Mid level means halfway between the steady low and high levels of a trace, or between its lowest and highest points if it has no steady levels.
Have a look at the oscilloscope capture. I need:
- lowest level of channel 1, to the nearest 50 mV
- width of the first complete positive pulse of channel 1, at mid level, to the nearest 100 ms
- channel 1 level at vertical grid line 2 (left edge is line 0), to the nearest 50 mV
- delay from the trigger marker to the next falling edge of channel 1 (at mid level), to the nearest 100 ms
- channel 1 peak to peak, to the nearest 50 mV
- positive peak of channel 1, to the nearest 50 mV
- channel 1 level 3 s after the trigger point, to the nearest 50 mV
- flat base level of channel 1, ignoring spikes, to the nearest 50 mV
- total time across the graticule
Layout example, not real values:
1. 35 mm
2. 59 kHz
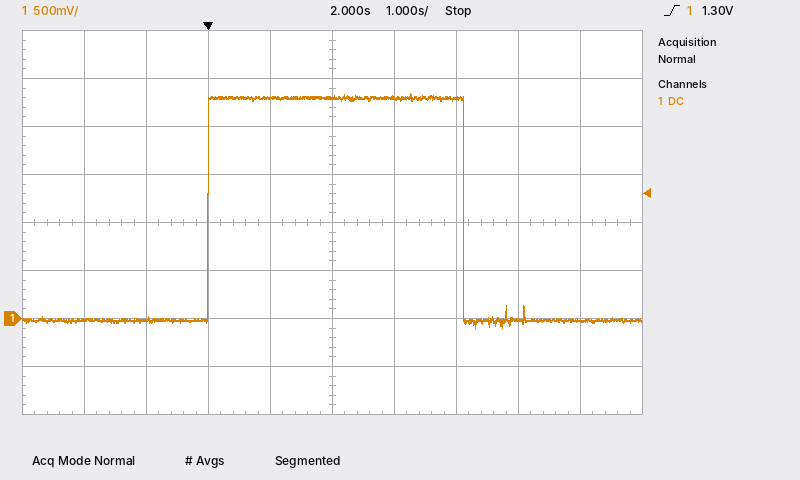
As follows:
1. -100 mV
2. 4.1 s
3. 0 mV
4. 4.1 s
5. 2.45 V
6. 2.35 V
7. 2.30 V
8. 0 mV
9. 10 s
